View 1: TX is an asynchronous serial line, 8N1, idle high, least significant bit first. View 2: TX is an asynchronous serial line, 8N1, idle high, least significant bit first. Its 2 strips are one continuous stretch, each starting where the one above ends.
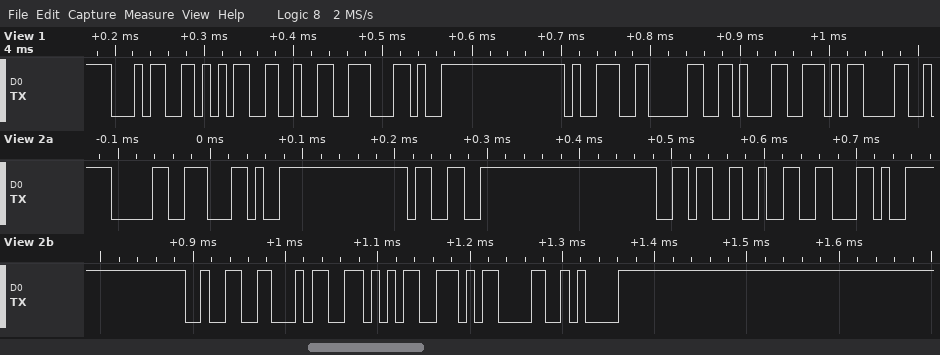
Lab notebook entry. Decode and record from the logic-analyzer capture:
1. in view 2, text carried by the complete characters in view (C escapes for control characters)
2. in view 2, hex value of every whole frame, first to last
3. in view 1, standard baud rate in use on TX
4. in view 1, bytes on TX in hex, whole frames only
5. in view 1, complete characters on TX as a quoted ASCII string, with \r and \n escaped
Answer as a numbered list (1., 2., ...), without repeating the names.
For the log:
1. "0,362,245\r\n"
2. 30 2C 33 36 32 2C 32 34 35 0D 0A
3. 115200 baud
4. 34 35 32 2C 39 30 31 0D
5. "452,901\r"
